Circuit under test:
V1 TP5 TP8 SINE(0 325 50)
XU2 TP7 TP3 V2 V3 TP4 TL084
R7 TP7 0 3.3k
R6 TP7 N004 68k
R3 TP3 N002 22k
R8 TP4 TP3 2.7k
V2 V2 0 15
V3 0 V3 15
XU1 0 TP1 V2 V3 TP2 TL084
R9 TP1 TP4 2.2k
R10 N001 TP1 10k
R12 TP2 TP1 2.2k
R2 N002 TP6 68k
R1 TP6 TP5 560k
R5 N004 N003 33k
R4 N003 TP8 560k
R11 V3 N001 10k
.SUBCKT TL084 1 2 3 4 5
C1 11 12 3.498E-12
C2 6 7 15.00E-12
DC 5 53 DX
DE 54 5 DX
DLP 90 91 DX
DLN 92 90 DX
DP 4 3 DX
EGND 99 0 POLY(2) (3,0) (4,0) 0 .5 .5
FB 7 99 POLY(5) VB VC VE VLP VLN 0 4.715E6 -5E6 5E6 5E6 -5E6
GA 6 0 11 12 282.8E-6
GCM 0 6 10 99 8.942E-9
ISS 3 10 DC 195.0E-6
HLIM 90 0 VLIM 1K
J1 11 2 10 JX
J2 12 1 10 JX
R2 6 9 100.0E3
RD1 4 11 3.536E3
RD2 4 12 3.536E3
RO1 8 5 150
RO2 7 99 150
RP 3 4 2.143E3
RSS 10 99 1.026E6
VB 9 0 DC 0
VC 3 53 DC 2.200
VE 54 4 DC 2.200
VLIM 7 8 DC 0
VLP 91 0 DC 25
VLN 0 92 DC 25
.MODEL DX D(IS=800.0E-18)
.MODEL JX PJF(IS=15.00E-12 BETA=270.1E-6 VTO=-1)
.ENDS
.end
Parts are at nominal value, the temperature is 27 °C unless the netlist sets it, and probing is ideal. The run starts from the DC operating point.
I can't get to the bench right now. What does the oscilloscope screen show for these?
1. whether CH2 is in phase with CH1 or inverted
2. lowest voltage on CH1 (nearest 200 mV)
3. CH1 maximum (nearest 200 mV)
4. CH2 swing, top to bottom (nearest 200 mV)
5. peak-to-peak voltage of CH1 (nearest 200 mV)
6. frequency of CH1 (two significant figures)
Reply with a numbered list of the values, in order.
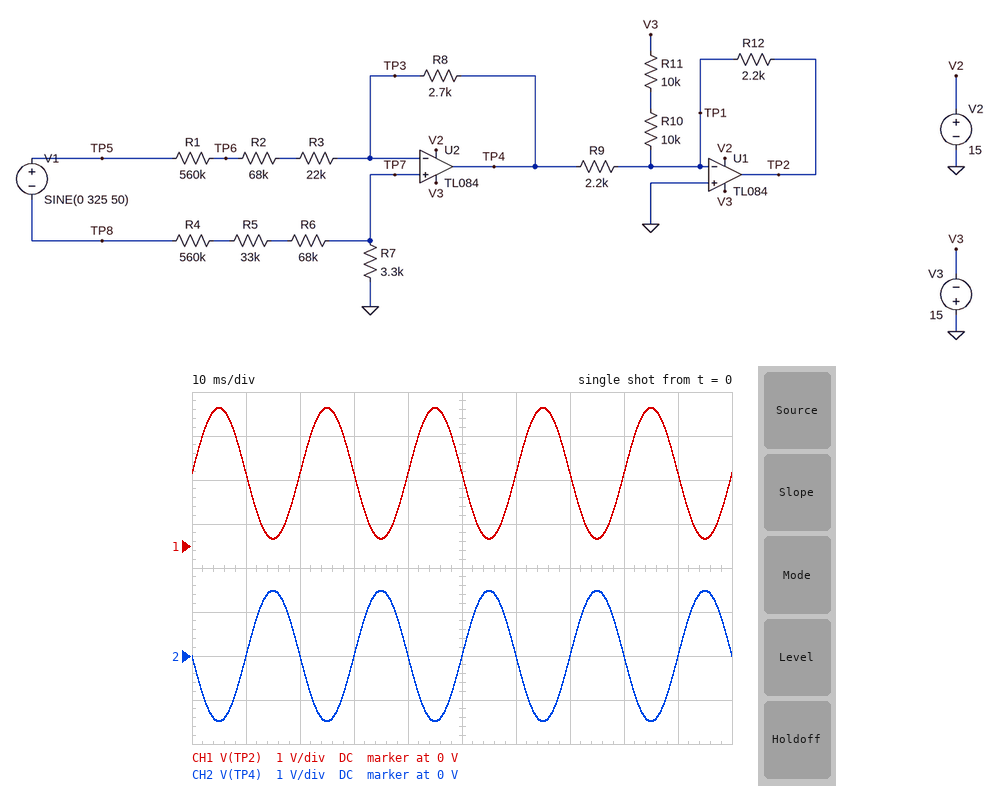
1. inverted
2. 200 mV
3. 3.2 V
4. 3.0 V
5. 3.0 V
6. 50 Hz
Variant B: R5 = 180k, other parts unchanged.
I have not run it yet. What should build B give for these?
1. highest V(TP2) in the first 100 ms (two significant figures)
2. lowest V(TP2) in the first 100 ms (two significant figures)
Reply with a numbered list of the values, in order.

1. 3.0 V
2. 310 mV
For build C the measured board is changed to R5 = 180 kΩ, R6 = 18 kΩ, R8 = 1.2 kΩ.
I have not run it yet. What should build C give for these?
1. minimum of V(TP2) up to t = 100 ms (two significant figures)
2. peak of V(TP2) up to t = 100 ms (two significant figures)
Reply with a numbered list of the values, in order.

1. 610 mV
2. 2.7 V
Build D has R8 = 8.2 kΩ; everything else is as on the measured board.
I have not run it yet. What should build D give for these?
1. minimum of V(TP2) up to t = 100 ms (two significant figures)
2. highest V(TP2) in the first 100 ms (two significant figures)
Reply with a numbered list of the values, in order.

1. -1.2 V
2. 4.5 V
